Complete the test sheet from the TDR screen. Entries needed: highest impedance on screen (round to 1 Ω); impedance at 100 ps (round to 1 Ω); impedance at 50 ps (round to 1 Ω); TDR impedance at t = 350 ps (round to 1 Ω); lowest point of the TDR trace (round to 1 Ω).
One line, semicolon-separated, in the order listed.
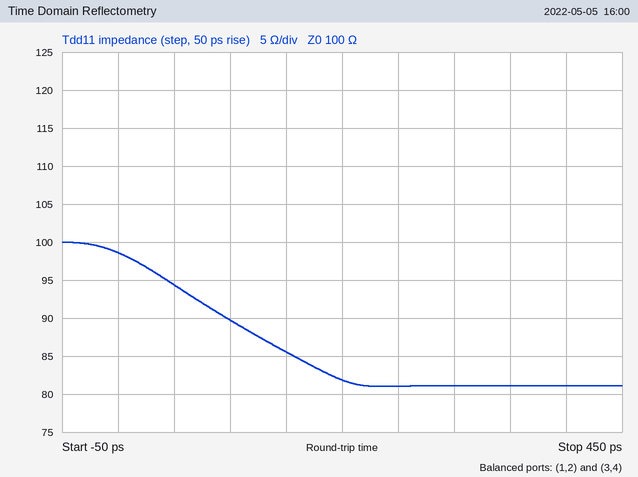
100 Ω; 90 Ω; 94 Ω; 81 Ω; 81 Ω
